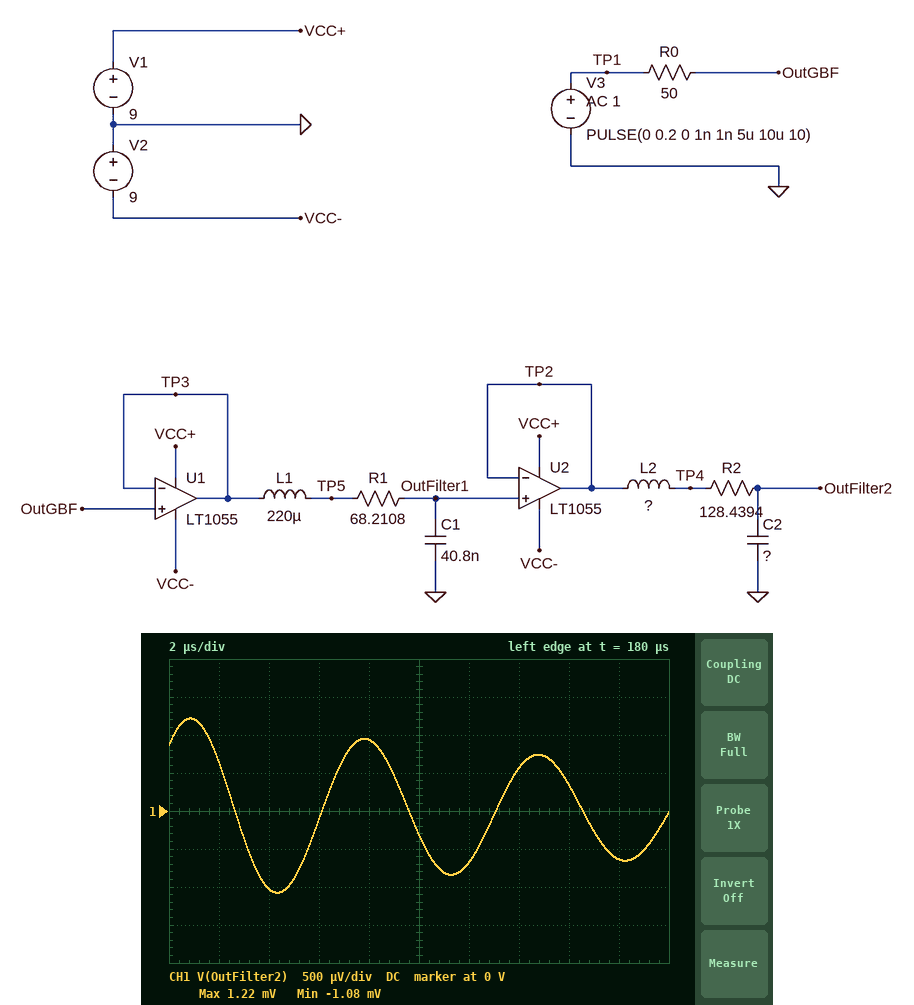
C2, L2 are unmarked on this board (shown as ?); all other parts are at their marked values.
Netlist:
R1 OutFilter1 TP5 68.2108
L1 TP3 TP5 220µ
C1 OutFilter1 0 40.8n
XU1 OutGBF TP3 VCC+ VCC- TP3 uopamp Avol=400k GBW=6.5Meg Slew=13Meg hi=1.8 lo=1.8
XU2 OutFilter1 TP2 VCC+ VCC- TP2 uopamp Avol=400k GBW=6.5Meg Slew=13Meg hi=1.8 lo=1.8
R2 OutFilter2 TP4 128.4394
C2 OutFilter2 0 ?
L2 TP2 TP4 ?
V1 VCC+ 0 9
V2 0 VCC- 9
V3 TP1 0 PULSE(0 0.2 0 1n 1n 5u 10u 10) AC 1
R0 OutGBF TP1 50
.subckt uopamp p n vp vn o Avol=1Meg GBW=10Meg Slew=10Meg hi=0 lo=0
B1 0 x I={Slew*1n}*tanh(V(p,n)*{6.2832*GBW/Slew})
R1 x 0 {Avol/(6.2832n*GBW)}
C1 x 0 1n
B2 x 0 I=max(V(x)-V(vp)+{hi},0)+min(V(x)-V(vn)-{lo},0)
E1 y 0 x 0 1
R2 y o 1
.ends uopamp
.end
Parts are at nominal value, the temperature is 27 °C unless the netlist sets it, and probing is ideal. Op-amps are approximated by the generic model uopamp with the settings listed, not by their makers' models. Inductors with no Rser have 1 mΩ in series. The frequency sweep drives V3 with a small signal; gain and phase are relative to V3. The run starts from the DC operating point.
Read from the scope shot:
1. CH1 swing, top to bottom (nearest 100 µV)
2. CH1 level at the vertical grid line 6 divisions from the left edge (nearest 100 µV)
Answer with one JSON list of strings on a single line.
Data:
["2.3 mV", "-700 µV"]
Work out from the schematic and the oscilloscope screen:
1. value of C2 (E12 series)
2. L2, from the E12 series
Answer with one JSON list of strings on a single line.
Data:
["680 pF", "1.8 mH"]
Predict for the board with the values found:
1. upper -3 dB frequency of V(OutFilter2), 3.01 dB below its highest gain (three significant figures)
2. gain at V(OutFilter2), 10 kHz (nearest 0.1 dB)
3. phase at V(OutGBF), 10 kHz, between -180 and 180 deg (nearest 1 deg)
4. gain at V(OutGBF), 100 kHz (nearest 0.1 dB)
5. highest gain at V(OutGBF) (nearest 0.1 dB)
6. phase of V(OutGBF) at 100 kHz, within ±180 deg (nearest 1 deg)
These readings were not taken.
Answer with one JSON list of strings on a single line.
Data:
["148 kHz", "0.2 dB", "0 deg", "0 dB", "0 dB", "0 deg"]
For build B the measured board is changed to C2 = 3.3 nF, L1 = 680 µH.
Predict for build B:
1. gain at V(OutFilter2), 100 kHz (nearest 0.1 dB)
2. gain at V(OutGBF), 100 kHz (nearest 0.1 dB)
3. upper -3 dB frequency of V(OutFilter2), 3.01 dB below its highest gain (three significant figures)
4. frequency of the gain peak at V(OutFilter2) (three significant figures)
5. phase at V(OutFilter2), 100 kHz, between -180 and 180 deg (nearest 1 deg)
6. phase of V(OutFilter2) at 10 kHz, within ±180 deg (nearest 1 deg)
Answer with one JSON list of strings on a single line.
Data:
["-22.8 dB", "0 dB", "37.8 kHz", "29.1 kHz", "19 deg", "-13 deg"]
